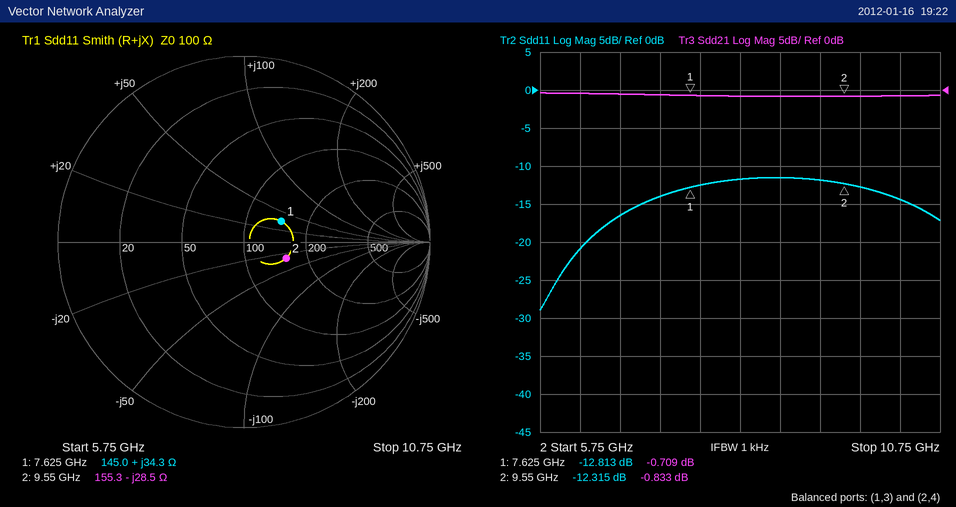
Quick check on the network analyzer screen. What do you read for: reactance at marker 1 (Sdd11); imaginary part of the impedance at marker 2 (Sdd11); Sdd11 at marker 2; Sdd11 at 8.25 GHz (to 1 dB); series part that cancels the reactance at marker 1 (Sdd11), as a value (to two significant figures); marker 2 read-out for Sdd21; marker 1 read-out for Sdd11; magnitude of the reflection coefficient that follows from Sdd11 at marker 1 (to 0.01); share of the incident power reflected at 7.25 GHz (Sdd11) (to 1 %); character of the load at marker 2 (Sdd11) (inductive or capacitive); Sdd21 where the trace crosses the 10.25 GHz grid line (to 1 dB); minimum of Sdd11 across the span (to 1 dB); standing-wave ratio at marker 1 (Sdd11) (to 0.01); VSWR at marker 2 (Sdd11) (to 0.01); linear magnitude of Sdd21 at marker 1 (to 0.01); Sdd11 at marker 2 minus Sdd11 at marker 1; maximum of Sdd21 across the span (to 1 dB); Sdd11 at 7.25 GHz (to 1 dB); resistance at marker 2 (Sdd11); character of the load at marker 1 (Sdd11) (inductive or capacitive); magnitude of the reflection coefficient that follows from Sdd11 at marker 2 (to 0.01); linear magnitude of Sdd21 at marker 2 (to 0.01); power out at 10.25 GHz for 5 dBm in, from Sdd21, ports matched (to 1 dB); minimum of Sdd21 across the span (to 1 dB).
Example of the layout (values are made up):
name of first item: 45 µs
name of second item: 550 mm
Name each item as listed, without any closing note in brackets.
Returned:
reactance at marker 1: +34.3 Ω
imaginary part of the impedance at marker 2: -28.5 Ω
Sdd11 at marker 2: -12.315 dB
Sdd11 at 8.25 GHz: -12 dB
series part that cancels the reactance at marker 1 (Sdd11), as a value: 610 fF
marker 2 read-out for Sdd21: -0.833 dB
marker 1 read-out for Sdd11: -12.813 dB
magnitude of the reflection coefficient that follows from Sdd11 at marker 1: 0.23
share of the incident power reflected at 7.25 GHz (Sdd11): 4 %
character of the load at marker 2 (Sdd11): capacitive
Sdd21 where the trace crosses the 10.25 GHz grid line: -1 dB
minimum of Sdd11 across the span: -29 dB
standing-wave ratio at marker 1 (Sdd11): 1.59
VSWR at marker 2 (Sdd11): 1.64
linear magnitude of Sdd21 at marker 1: 0.92
Sdd11 at marker 2 minus Sdd11 at marker 1: 0.498 dB
maximum of Sdd21 across the span: 0 dB
Sdd11 at 7.25 GHz: -14 dB
resistance at marker 2: 155.3 Ω
character of the load at marker 1 (Sdd11): inductive
magnitude of the reflection coefficient that follows from Sdd11 at marker 2: 0.24
linear magnitude of Sdd21 at marker 2: 0.91
power out at 10.25 GHz for 5 dBm in, from Sdd21, ports matched: 4 dBm
minimum of Sdd21 across the span: -1 dB
